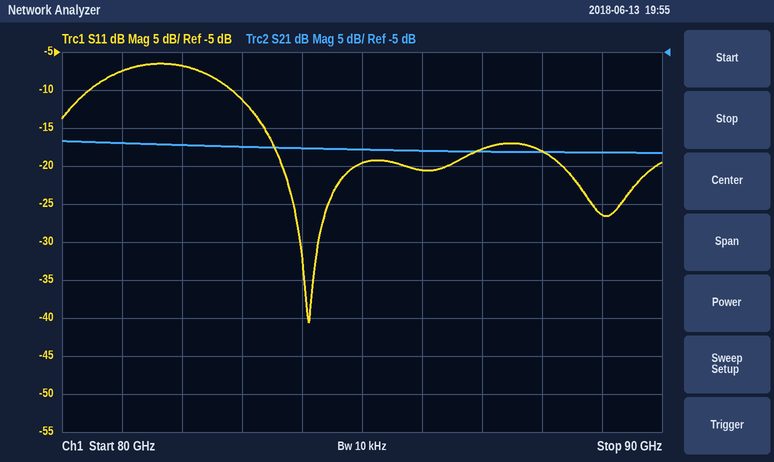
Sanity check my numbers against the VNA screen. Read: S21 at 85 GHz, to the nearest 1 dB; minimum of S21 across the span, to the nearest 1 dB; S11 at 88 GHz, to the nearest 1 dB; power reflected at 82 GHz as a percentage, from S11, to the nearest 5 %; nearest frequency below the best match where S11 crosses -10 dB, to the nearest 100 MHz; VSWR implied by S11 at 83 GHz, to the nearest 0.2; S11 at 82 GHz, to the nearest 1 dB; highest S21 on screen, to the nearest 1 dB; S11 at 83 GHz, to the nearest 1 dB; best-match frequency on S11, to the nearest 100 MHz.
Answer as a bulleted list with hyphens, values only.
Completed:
- -18 dB
- -18 dB
- -18 dB
- 20 %
- 82.8 GHz
- 1.8
- -7 dB
- -17 dB
- -11 dB
- 84.1 GHz
